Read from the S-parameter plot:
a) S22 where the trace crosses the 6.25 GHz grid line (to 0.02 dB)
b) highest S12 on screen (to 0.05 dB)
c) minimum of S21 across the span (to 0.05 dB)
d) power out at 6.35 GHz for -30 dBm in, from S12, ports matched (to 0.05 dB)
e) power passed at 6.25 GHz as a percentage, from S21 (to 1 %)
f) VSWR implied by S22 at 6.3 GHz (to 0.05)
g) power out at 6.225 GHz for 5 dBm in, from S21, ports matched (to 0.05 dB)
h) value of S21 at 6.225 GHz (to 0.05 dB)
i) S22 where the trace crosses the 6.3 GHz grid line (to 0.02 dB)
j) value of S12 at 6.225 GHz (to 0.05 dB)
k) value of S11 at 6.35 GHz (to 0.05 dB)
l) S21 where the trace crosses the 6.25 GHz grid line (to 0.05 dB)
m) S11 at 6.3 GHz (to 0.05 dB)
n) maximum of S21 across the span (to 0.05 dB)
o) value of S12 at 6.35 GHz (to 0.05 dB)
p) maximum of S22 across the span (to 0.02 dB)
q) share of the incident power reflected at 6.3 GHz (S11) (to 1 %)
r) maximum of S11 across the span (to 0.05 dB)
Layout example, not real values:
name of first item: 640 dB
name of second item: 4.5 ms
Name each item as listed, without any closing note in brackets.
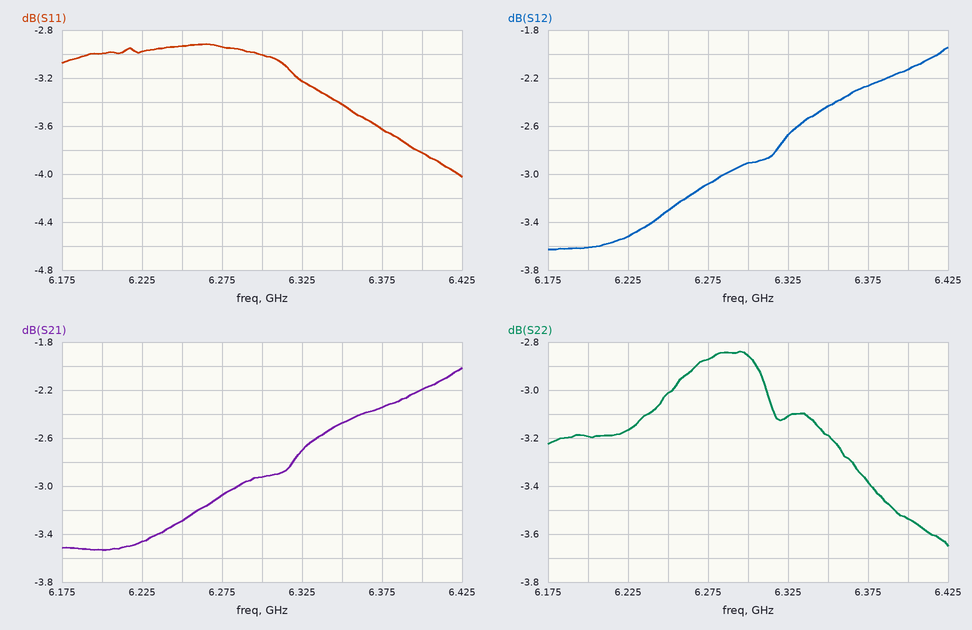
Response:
S22 where the trace crosses the 6.25 GHz grid line: -3.02 dB
highest S12 on screen: -1.95 dB
minimum of S21 across the span: -3.55 dB
power out at 6.35 GHz for -30 dBm in, from S12, ports matched: -32.45 dBm
power passed at 6.25 GHz as a percentage, from S21: 47 %
VSWR implied by S22 at 6.3 GHz: 6.15
power out at 6.225 GHz for 5 dBm in, from S21, ports matched: 1.55 dBm
value of S21 at 6.225 GHz: -3.45 dB
S22 where the trace crosses the 6.3 GHz grid line: -2.86 dB
value of S12 at 6.225 GHz: -3.50 dB
value of S11 at 6.35 GHz: -3.40 dB
S21 where the trace crosses the 6.25 GHz grid line: -3.30 dB
S11 at 6.3 GHz: -3.00 dB
maximum of S21 across the span: -2.00 dB
value of S12 at 6.35 GHz: -2.45 dB
maximum of S22 across the span: -2.84 dB
share of the incident power reflected at 6.3 GHz (S11): 50 %
maximum of S11 across the span: -2.90 dB
